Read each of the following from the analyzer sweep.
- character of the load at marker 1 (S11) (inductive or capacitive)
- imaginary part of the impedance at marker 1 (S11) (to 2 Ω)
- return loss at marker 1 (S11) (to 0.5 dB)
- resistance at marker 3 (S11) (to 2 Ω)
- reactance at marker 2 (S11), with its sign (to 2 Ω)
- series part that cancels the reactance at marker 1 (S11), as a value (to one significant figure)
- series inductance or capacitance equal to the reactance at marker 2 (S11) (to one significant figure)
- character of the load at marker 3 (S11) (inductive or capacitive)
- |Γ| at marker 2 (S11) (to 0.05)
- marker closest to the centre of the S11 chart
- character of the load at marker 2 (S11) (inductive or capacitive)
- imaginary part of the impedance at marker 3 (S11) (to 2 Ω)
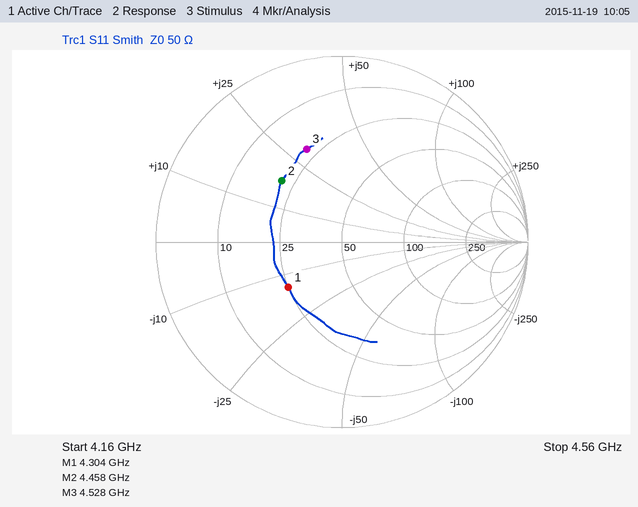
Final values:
capacitive
-14 Ω
8.5 dB
22 Ω
+18 Ω
500 pH
600 pH
inductive
0.45
marker 1
inductive
+30 Ω
